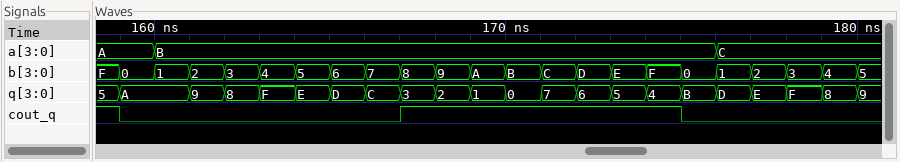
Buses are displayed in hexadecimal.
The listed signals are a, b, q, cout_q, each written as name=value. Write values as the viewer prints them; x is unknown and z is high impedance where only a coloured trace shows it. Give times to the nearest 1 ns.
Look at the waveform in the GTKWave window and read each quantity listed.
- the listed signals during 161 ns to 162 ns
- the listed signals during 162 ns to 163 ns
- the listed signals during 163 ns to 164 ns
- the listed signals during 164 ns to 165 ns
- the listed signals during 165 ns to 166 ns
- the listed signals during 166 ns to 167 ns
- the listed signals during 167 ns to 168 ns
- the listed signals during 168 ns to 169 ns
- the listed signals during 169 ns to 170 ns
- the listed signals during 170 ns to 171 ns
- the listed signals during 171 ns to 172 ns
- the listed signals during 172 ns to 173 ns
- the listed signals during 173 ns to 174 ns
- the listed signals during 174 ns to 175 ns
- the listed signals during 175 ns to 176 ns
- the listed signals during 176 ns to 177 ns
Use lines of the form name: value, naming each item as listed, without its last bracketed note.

the listed signals during 161 ns to 162 ns: a=B, b=2, q=9, cout_q=0
the listed signals during 162 ns to 163 ns: a=B, b=3, q=8, cout_q=0
the listed signals during 163 ns to 164 ns: a=B, b=4, q=F, cout_q=0
the listed signals during 164 ns to 165 ns: a=B, b=5, q=E, cout_q=0
the listed signals during 165 ns to 166 ns: a=B, b=6, q=D, cout_q=0
the listed signals during 166 ns to 167 ns: a=B, b=7, q=C, cout_q=0
the listed signals during 167 ns to 168 ns: a=B, b=8, q=3, cout_q=1
the listed signals during 168 ns to 169 ns: a=B, b=9, q=2, cout_q=1
the listed signals during 169 ns to 170 ns: a=B, b=A, q=1, cout_q=1
the listed signals during 170 ns to 171 ns: a=B, b=B, q=0, cout_q=1
the listed signals during 171 ns to 172 ns: a=B, b=C, q=7, cout_q=1
the listed signals during 172 ns to 173 ns: a=B, b=D, q=6, cout_q=1
the listed signals during 173 ns to 174 ns: a=B, b=E, q=5, cout_q=1
the listed signals during 174 ns to 175 ns: a=B, b=F, q=4, cout_q=1
the listed signals during 175 ns to 176 ns: a=B, b=0, q=B, cout_q=0
the listed signals during 176 ns to 177 ns: a=C, b=1, q=D, cout_q=0
